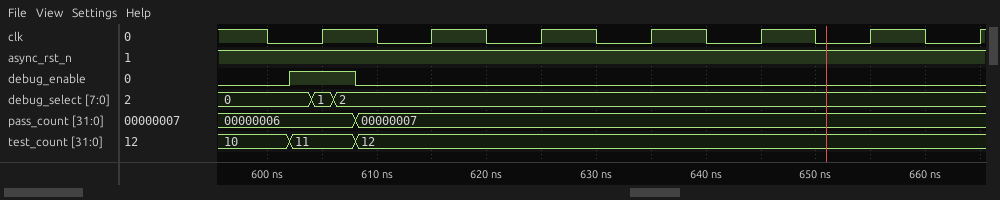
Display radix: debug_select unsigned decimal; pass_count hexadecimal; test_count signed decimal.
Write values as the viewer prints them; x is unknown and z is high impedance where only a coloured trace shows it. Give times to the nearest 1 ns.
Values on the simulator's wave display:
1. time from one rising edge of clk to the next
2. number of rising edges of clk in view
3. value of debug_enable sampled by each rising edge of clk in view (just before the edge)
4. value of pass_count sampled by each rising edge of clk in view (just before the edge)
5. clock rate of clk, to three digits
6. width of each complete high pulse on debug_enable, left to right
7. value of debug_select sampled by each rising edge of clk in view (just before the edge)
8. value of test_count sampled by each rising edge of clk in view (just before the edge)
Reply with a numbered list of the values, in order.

1. 10 ns
2. 7
3. 1 0 0 0 0 0 0
4. 00000006, 00000007, 00000007, 00000007, 00000007, 00000007, 00000007
5. 100 MHz
6. 6 ns
7. 1, 2, 2, 2, 2, 2, 2
8. 11, 12, 12, 12, 12, 12, 12
